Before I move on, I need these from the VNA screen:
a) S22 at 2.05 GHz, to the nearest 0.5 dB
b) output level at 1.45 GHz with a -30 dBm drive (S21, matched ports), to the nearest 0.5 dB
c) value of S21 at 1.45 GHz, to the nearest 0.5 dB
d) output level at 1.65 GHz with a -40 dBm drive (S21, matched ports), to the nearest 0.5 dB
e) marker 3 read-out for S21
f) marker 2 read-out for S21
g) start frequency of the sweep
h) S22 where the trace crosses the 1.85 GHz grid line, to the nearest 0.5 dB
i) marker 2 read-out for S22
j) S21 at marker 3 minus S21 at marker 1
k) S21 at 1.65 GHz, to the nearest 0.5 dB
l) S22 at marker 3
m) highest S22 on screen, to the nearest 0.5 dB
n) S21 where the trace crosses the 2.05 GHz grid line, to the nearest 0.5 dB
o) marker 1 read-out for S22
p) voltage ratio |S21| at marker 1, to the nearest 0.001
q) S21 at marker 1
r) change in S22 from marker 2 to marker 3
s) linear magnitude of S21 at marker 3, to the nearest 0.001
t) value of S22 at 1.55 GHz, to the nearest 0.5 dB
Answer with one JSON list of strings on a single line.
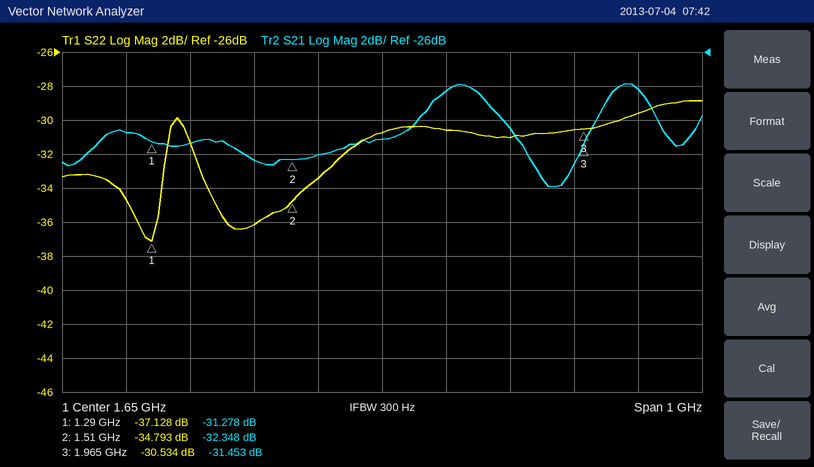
["-29.5 dB", "-62.5 dBm", "-32.5 dB", "-71.0 dBm", "-31.453 dB", "-32.348 dB", "1.15 GHz", "-31.0 dB", "-34.793 dB", "-0.175 dB", "-31.0 dB", "-30.534 dB", "-29.0 dB", "-28.0 dB", "-37.128 dB", "0.027", "-31.278 dB", "4.259 dB", "0.027", "-33.5 dB"]
